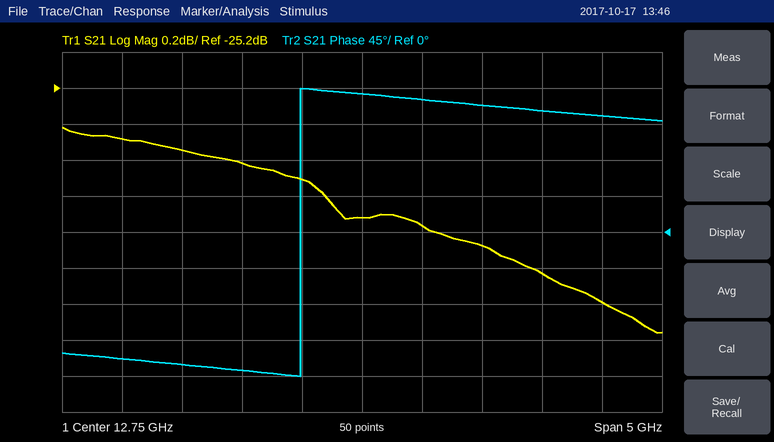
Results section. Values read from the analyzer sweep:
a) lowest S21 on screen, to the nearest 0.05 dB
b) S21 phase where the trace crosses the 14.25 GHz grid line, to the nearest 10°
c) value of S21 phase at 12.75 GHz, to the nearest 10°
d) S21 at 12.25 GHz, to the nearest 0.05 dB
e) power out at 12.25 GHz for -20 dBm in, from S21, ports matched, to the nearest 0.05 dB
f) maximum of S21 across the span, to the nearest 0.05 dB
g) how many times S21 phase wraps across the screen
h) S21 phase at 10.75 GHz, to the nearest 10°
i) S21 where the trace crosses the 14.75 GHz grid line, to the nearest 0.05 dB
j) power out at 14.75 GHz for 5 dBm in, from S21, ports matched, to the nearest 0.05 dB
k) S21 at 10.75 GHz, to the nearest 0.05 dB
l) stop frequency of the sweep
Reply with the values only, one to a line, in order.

-26.55 dB
150°
170°
-25.70 dB
-45.70 dBm
-25.40 dB
1
-160°
-26.40 dB
-21.40 dBm
-25.50 dB
15.25 GHz
